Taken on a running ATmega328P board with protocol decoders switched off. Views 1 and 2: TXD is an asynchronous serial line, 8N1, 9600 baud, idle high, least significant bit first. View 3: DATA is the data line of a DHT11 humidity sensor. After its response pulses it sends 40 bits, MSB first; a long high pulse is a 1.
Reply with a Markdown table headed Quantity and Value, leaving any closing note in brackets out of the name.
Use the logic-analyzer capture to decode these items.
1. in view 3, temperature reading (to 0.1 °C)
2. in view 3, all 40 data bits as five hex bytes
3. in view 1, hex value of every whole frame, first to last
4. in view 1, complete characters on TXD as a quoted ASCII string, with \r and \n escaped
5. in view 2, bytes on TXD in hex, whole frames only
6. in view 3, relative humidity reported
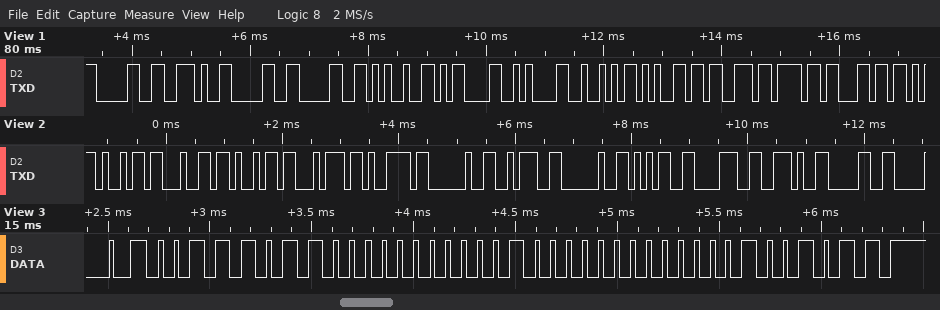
| Quantity | Value |
|---|---|
| in view 3, temperature reading | 16.0 °C |
| in view 3, all 40 data bits as five hex bytes | 3B 00 10 00 4B |
| in view 1, hex value of every whole frame, first to last | 30 2E 30 30 25 0D 0A 52 65 73 6F 6C |
| in view 1, complete characters on TXD as a quoted ASCII string, with \r and \n escaped | "0.00%\r\nResol" |
| in view 2, bytes on TXD in hex, whole frames only | 69 64 69 74 79 20 3A 20 35 38 2E 30 |
| in view 3, relative humidity reported | 59 % |
